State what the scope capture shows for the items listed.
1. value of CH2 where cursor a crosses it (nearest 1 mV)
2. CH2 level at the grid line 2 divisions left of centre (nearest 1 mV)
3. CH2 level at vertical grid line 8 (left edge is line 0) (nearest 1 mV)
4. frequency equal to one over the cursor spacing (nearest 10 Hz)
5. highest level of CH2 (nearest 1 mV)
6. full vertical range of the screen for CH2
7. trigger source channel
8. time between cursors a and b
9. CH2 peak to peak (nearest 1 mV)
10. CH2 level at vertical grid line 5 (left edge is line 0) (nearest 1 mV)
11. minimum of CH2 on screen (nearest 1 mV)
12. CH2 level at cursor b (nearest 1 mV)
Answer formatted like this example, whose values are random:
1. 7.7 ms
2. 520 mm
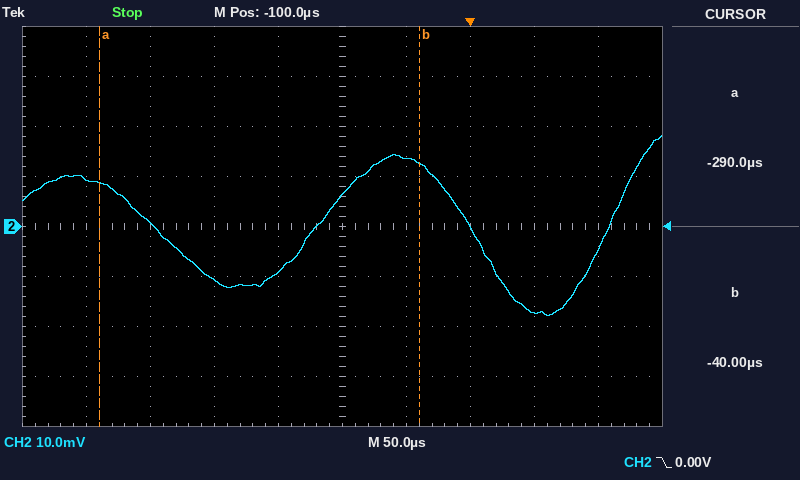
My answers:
1. 9 mV
2. -11 mV
3. -17 mV
4. 4.00 kHz
5. 18 mV
6. 80 mV
7. CH2
8. 250 µs
9. 36 mV
10. 6 mV
11. -18 mV
12. 13 mV
